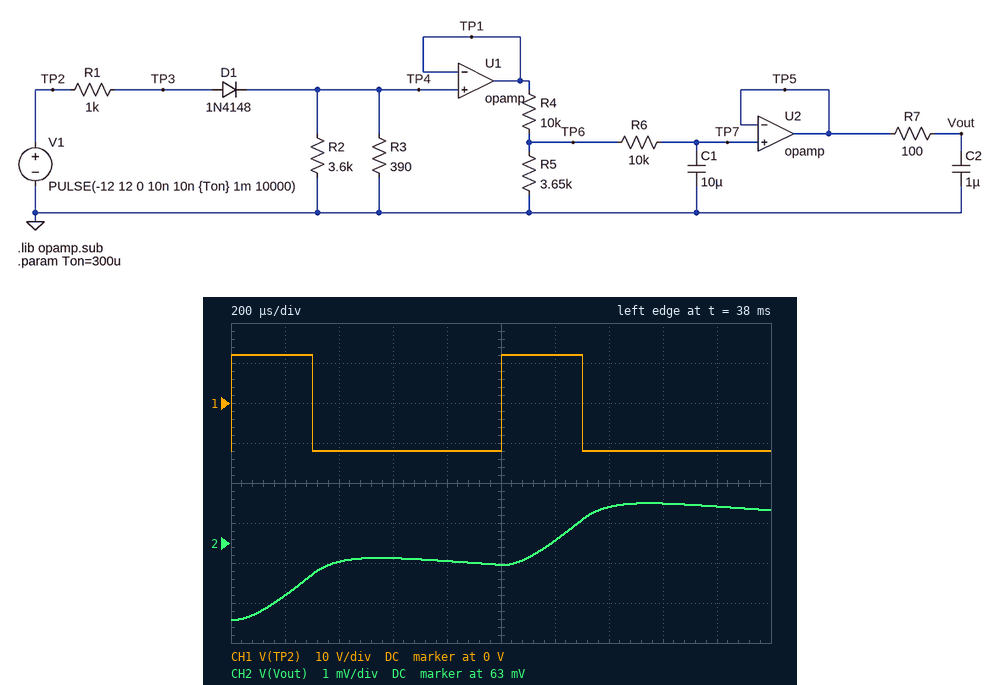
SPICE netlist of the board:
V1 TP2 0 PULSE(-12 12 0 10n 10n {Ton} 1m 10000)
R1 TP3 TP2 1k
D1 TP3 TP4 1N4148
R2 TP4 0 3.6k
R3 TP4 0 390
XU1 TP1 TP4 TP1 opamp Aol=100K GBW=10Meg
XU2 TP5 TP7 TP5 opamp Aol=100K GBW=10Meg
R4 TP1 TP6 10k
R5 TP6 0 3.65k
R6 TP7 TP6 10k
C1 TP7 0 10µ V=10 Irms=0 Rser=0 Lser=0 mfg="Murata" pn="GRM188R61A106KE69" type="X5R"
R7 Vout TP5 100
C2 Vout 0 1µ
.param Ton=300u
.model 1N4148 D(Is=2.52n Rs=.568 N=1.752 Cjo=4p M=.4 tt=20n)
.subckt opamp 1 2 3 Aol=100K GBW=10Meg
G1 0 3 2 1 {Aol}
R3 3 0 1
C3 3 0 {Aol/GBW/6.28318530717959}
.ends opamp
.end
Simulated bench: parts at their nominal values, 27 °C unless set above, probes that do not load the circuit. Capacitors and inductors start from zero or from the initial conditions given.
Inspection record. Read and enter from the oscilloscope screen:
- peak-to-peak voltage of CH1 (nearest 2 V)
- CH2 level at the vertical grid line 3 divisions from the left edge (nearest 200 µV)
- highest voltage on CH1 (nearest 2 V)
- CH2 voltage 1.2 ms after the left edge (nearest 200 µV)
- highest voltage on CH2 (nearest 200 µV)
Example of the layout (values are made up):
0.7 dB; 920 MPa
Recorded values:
24 V; 62.6 mV; 12 V; 63.0 mV; 64.0 mV
